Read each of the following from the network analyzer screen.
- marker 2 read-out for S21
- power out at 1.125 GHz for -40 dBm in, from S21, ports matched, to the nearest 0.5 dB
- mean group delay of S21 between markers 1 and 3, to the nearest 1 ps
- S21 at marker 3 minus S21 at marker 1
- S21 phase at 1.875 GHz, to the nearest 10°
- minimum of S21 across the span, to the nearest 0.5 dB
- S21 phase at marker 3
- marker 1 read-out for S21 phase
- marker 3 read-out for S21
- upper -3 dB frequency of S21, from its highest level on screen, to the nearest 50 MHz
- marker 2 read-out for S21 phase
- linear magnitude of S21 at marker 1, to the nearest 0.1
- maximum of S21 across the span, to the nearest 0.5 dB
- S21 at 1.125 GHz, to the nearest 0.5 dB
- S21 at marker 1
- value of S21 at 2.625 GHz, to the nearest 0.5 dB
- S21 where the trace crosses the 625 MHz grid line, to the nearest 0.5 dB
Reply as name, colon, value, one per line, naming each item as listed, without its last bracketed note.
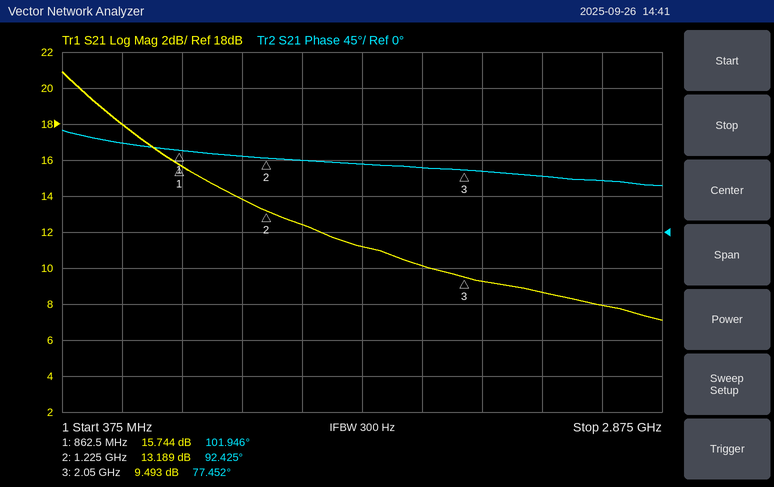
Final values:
marker 2 read-out for S21: 13.189 dB
power out at 1.125 GHz for -40 dBm in, from S21, ports matched, to the nearest 0.5 dB: -26.0 dBm
mean group delay of S21 between markers 1 and 3, to the nearest 1 ps: 57 ps
S21 at marker 3 minus S21 at marker 1: -6.251 dB
S21 phase at 1.875 GHz, to the nearest 10°: 80°
minimum of S21 across the span, to the nearest 0.5 dB: 7.0 dB
S21 phase at marker 3: 77.452°
marker 1 read-out for S21 phase: 101.946°
marker 3 read-out for S21: 9.493 dB
upper -3 dB frequency of S21, from its highest level on screen, to the nearest 50 MHz: 650 MHz
marker 2 read-out for S21 phase: 92.425°
linear magnitude of S21 at marker 1, to the nearest 0.1: 6.1
maximum of S21 across the span, to the nearest 0.5 dB: 21.0 dB
S21 at 1.125 GHz, to the nearest 0.5 dB: 14.0 dB
S21 at marker 1: 15.744 dB
value of S21 at 2.625 GHz, to the nearest 0.5 dB: 8.0 dB
S21 where the trace crosses the 625 MHz grid line, to the nearest 0.5 dB: 18.0 dB
